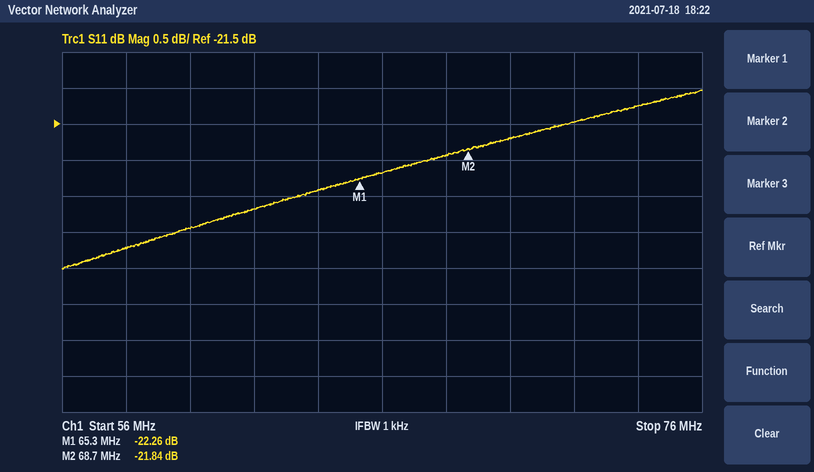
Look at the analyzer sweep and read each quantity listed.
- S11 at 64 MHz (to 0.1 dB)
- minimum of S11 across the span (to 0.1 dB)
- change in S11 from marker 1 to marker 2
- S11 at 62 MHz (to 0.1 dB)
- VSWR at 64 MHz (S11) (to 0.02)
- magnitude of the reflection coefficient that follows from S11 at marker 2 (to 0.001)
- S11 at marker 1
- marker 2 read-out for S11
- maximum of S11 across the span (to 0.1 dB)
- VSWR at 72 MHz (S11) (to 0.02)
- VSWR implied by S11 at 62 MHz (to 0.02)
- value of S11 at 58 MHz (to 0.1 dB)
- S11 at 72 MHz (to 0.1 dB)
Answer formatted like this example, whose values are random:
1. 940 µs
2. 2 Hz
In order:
1. -22.4 dB
2. -23.5 dB
3. 0.42 dB
4. -22.7 dB
5. 1.16
6. 0.081
7. -22.26 dB
8. -21.84 dB
9. -21.0 dB
10. 1.18
11. 1.16
12. -23.2 dB
13. -21.5 dB
